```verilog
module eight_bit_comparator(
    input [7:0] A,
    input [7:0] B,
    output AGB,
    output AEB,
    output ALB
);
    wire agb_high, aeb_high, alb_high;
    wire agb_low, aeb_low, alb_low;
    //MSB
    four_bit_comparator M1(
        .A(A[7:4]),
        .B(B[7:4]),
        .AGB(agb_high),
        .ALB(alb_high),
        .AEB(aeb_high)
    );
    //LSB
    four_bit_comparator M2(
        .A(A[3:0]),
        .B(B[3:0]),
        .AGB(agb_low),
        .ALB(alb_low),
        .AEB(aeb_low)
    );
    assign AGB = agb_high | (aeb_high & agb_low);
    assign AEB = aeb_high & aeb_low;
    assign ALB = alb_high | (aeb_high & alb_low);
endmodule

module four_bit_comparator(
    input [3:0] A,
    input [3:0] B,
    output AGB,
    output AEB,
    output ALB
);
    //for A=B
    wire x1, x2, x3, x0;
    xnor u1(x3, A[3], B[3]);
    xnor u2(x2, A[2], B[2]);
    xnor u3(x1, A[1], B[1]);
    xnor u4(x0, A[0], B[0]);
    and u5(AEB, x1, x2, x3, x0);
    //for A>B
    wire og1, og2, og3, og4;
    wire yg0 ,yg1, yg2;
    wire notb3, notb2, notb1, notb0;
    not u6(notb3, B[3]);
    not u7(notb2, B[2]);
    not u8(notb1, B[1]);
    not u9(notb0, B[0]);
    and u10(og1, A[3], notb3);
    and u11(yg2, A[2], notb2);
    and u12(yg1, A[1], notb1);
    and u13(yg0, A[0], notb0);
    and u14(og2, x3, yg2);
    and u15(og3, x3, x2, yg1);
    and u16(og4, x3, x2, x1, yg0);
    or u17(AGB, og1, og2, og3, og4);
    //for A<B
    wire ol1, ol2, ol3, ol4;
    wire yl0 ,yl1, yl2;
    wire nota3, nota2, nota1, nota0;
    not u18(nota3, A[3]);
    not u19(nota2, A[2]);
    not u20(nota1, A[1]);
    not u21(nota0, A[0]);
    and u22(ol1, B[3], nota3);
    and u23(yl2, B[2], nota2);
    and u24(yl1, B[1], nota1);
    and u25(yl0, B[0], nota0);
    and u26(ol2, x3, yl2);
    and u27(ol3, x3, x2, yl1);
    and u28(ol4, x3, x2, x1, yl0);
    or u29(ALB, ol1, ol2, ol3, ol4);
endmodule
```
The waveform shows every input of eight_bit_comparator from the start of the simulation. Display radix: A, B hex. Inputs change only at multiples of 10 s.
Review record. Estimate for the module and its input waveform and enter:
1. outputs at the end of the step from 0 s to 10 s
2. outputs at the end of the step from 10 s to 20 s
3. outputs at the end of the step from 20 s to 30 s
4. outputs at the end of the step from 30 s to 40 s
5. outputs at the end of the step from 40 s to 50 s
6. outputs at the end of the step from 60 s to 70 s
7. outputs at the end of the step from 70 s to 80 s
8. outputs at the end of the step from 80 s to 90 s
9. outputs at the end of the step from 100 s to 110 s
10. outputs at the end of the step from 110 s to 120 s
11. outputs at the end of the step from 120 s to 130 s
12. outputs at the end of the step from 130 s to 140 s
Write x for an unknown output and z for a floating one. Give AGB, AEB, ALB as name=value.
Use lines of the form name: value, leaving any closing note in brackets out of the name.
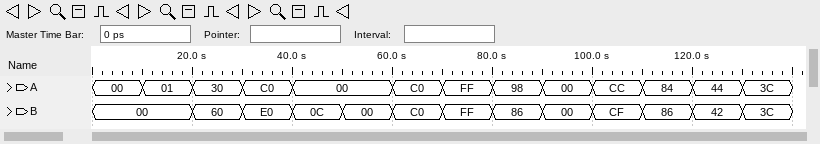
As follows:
outputs at the end of the step from 0 s to 10 s: AGB=0, AEB=1, ALB=0
outputs at the end of the step from 10 s to 20 s: AGB=1, AEB=0, ALB=0
outputs at the end of the step from 20 s to 30 s: AGB=0, AEB=0, ALB=1
outputs at the end of the step from 30 s to 40 s: AGB=0, AEB=0, ALB=1
outputs at the end of the step from 40 s to 50 s: AGB=0, AEB=0, ALB=1
outputs at the end of the step from 60 s to 70 s: AGB=0, AEB=1, ALB=0
outputs at the end of the step from 70 s to 80 s: AGB=0, AEB=1, ALB=0
outputs at the end of the step from 80 s to 90 s: AGB=1, AEB=0, ALB=0
outputs at the end of the step from 100 s to 110 s: AGB=0, AEB=0, ALB=1
outputs at the end of the step from 110 s to 120 s: AGB=0, AEB=0, ALB=1
outputs at the end of the step from 120 s to 130 s: AGB=1, AEB=0, ALB=0
outputs at the end of the step from 130 s to 140 s: AGB=0, AEB=1, ALB=0
